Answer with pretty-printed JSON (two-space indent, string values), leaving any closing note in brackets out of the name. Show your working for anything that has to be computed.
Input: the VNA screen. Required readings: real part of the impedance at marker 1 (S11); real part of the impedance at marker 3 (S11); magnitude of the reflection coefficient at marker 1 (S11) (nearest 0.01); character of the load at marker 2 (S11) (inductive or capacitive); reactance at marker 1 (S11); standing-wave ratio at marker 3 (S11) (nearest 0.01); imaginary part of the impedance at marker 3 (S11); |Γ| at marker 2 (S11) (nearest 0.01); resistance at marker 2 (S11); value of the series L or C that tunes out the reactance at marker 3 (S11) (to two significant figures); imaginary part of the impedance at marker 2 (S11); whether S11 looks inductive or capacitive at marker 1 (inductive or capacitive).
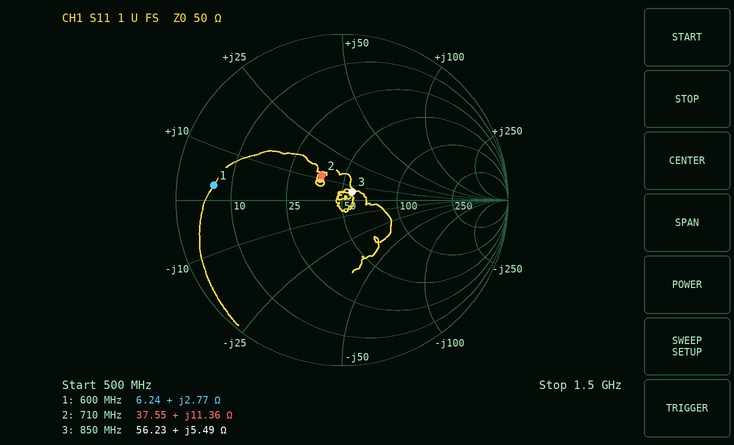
{
  "real part of the impedance at marker 1": "6.24 Ω",
  "real part of the impedance at marker 3": "56.23 Ω",
  "magnitude of the reflection coefficient at marker 1 (S11)": "0.78",
  "character of the load at marker 2 (S11)": "inductive",
  "reactance at marker 1": "+2.77 Ω",
  "standing-wave ratio at marker 3 (S11)": "1.17",
  "imaginary part of the impedance at marker 3": "+5.49 Ω",
  "|Γ| at marker 2 (S11)": "0.19",
  "resistance at marker 2": "37.55 Ω",
  "value of the series L or C that tunes out the reactance at marker 3 (S11)": "C = 1/(2π × 850 MHz × 5.49 Ω) ≈ 34 pF",
  "imaginary part of the impedance at marker 2": "+11.36 Ω",
  "whether S11 looks inductive or capacitive at marker 1": "inductive"
}
